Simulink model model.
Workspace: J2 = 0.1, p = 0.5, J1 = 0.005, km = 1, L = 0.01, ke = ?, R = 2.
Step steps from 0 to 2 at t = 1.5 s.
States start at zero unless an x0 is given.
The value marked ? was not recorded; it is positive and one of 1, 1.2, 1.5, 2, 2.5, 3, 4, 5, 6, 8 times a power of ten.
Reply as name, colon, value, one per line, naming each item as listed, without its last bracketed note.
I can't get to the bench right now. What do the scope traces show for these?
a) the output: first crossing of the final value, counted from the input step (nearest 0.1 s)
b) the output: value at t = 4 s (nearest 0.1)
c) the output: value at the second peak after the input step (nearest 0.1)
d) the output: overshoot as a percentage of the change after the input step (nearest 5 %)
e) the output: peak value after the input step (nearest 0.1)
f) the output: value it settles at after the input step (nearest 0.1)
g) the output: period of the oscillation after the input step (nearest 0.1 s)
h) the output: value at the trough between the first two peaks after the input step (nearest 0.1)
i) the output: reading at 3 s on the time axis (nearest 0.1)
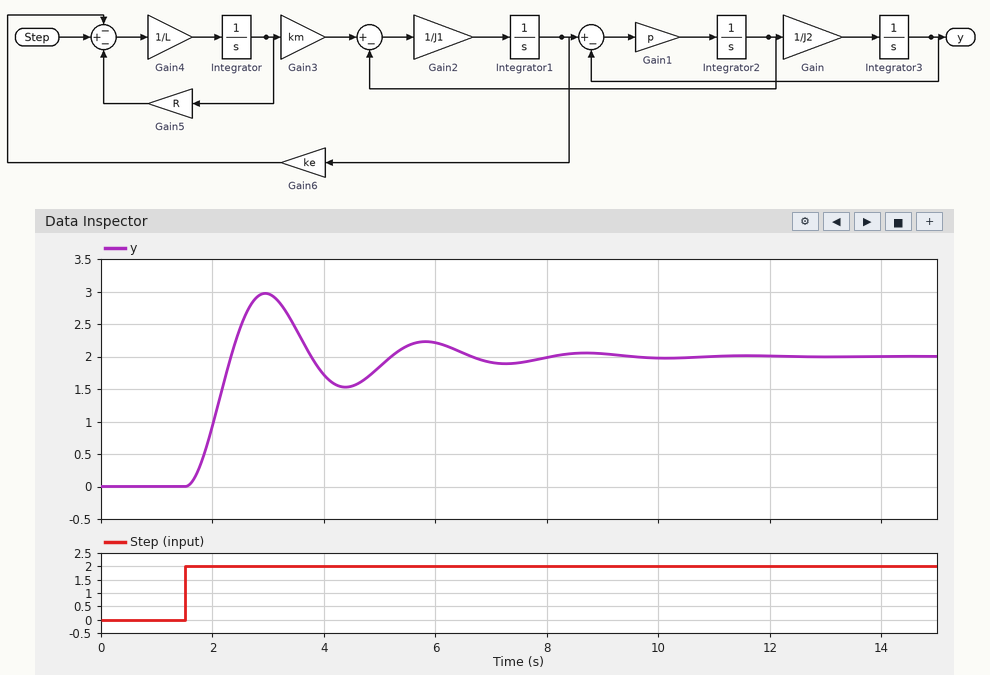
the output: first crossing of the final value, counted from the input step: 0.8 s
the output: value at t = 4 s: 1.7
the output: value at the second peak after the input step: 2.2
the output: overshoot as a percentage of the change after the input step: 50 %
the output: peak value after the input step: 3.0
the output: value it settles at after the input step: 2.0
the output: period of the oscillation after the input step: 2.9 s
the output: value at the trough between the first two peaks after the input step: 1.5
the output: reading at 3 s on the time axis: 3.0
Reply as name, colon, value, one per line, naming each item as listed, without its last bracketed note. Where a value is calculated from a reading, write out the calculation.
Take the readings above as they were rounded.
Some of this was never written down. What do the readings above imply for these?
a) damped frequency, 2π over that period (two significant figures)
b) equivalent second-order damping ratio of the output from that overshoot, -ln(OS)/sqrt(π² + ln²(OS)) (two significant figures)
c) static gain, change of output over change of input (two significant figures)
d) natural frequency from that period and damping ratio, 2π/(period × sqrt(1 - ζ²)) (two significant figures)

damped frequency, 2π over that period: 2π / 2.9 = 2.2 rad/s
equivalent second-order damping ratio of the output from that overshoot, -ln(OS)/sqrt(π² + ln²(OS)): ln(0.5) = -0.693; 0.693 / sqrt(9.870 + 0.480) = 0.22
static gain, change of output over change of input: (2 - 0) / (2 - 0) = 1.0
natural frequency from that period and damping ratio, 2π/(period × sqrt(1 - ζ²)): 2π / (2.9 × sqrt(1 - 0.22²)) = 2.2 rad/s
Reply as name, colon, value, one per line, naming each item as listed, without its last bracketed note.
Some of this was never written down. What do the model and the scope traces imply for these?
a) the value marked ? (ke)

the value marked ?: 1
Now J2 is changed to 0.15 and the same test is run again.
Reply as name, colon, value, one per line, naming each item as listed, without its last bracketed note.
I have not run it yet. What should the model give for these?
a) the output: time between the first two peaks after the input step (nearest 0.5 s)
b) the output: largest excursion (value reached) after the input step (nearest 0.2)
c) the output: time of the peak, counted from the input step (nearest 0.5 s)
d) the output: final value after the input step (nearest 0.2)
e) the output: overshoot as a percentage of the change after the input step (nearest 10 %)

the output: time between the first two peaks after the input step: 3.5 s
the output: largest excursion (value reached) after the input step: 2.8
the output: time of the peak, counted from the input step: 2.0 s
the output: final value after the input step: 2.0
the output: overshoot as a percentage of the change after the input step: 40 %
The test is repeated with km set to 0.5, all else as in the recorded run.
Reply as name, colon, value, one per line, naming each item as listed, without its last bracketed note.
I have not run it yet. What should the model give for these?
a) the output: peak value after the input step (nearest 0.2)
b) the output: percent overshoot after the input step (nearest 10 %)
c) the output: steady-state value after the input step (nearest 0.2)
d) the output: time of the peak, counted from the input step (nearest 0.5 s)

the output: peak value after the input step: 2.4
the output: percent overshoot after the input step: 20 %
the output: steady-state value after the input step: 2.0
the output: time of the peak, counted from the input step: 1.5 s
